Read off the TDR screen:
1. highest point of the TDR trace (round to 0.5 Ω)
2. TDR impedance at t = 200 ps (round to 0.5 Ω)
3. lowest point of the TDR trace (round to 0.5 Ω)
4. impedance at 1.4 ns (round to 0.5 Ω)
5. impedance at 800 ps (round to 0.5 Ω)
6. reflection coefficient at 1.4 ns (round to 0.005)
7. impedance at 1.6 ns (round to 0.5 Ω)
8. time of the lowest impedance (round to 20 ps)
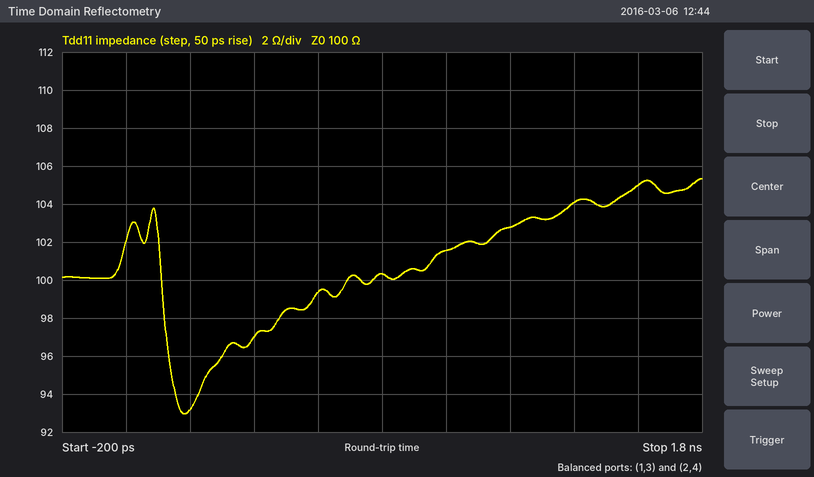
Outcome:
105.5 Ω
93.0 Ω
93.0 Ω
104.0 Ω
100.5 Ω
+0.020
105.0 Ω
180 ps
